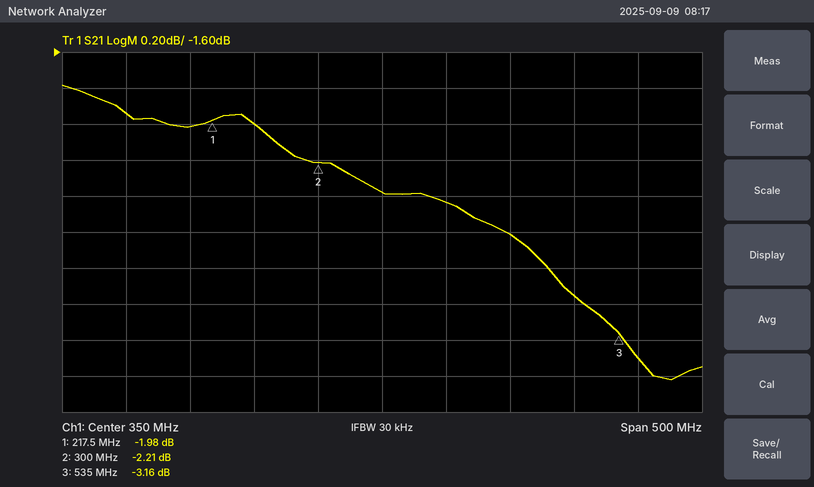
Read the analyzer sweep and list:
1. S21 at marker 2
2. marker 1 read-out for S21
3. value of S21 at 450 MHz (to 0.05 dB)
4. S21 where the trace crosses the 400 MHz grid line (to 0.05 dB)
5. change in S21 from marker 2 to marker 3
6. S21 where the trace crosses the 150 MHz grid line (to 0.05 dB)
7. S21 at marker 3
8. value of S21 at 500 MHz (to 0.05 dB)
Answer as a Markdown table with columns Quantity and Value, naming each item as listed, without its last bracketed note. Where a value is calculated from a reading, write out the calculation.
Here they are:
| Quantity | Value |
|---|---|
| S21 at marker 2 | -2.21 dB |
| marker 1 read-out for S21 | -1.98 dB |
| value of S21 at 450 MHz | -2.60 dB |
| S21 where the trace crosses the 400 MHz grid line | -2.45 dB |
| change in S21 from marker 2 to marker 3 | -3.16 − (-2.21) = -0.95 dB |
| S21 where the trace crosses the 150 MHz grid line | -1.95 dB |
| S21 at marker 3 | -3.16 dB |
| value of S21 at 500 MHz | -2.95 dB |
